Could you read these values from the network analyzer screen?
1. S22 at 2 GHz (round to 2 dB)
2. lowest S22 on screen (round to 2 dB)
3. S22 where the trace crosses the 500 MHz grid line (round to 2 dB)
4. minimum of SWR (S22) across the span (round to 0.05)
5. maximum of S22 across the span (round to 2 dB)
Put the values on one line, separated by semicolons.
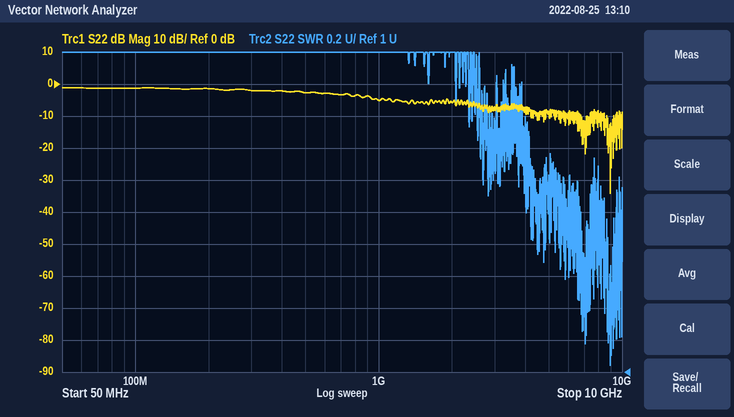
-6 dB; -34 dB; -2 dB; 1.05; -2 dB
